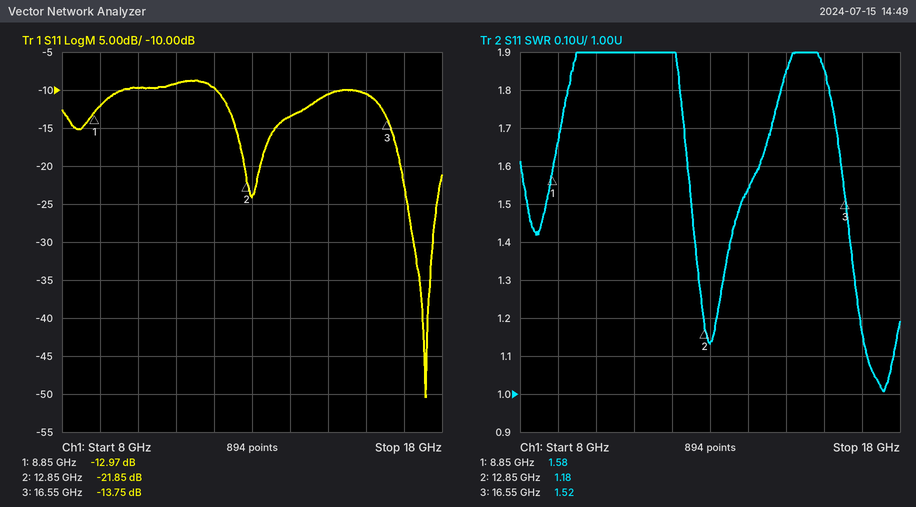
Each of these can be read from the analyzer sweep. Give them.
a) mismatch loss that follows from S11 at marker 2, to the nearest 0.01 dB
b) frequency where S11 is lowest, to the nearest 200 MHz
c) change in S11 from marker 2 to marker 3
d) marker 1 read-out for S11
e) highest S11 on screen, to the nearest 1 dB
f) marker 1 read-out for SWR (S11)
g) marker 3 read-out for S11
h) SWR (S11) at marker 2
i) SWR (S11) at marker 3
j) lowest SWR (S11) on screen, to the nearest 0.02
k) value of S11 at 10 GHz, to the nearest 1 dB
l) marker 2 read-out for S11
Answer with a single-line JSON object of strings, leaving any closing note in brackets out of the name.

{"mismatch loss that follows from S11 at marker 2, to the nearest 0.01 dB": "0.03 dB", "frequency where S11 is lowest, to the nearest 200 MHz": "17.6 GHz", "change in S11 from marker 2 to marker 3": "8.10 dB", "marker 1 read-out for S11": "-12.97 dB", "highest S11 on screen, to the nearest 1 dB": "-9 dB", "marker 1 read-out for SWR": "1.58", "marker 3 read-out for S11": "-13.75 dB", "SWR (S11) at marker 2": "1.18", "SWR (S11) at marker 3": "1.52", "lowest SWR (S11) on screen, to the nearest 0.02": "1.00", "value of S11 at 10 GHz, to the nearest 1 dB": "-10 dB", "marker 2 read-out for S11": "-21.85 dB"}
